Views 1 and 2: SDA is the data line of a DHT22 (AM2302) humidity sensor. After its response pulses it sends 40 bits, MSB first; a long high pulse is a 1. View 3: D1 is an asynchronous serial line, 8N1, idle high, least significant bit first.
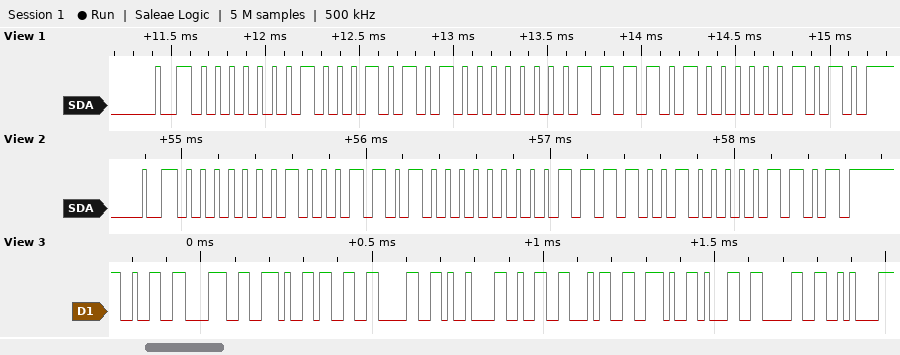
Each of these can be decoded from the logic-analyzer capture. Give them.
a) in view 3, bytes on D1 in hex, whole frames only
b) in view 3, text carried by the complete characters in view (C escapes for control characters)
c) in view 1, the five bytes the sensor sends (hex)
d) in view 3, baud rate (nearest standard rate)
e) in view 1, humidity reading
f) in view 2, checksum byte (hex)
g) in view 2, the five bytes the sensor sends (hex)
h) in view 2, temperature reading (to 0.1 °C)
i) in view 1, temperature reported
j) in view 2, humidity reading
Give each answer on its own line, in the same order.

32 38 2E 33 30 09 32 34 2E 31 30 0A
"28.30\t24.10\n"
01 15 00 F4 0A
57600 baud
27.7 %
0x0D
01 1A 00 F2 0D
24.2 °C
24.4 °C
28.2 %
